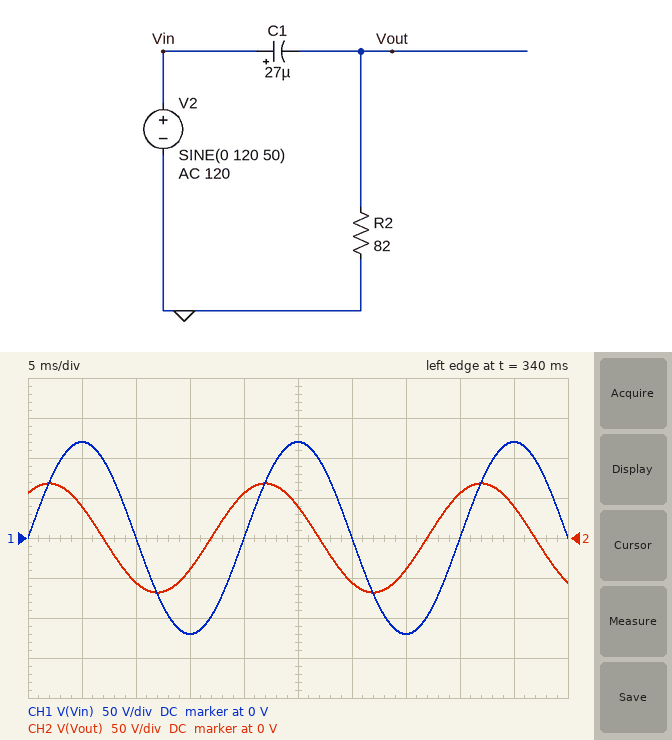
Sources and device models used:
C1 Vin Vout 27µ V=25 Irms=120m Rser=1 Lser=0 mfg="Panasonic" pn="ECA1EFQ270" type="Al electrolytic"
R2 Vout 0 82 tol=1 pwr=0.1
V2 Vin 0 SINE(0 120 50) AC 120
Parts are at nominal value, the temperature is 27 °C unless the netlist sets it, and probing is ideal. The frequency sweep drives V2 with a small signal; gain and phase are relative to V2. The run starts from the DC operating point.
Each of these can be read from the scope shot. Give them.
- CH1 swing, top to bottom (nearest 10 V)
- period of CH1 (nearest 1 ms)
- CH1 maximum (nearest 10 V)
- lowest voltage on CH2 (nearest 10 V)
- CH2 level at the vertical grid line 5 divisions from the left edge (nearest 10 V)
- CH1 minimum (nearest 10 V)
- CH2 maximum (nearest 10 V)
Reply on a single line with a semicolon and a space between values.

240 V; 20 ms; 120 V; -70 V; 40 V; -120 V; 70 V
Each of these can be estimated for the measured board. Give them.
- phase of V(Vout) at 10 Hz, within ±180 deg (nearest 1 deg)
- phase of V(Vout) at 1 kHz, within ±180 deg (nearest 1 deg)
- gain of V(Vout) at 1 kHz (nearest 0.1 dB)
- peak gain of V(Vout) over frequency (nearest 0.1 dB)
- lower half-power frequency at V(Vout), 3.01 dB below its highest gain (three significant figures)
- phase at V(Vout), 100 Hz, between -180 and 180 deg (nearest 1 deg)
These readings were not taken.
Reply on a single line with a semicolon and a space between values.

82 deg; 4 deg; -0.1 dB; -0.1 dB; 71.0 Hz; 35 deg
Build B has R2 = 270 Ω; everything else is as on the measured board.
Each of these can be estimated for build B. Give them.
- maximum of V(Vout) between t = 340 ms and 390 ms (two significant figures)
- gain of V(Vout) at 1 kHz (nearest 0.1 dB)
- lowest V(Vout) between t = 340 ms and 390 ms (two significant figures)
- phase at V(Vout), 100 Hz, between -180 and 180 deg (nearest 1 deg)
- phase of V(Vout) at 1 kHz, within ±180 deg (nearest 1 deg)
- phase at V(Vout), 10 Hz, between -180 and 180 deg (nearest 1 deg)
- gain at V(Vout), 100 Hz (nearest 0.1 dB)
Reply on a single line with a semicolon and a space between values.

110 V; 0 dB; -110 V; 12 deg; 1 deg; 65 deg; -0.2 dB
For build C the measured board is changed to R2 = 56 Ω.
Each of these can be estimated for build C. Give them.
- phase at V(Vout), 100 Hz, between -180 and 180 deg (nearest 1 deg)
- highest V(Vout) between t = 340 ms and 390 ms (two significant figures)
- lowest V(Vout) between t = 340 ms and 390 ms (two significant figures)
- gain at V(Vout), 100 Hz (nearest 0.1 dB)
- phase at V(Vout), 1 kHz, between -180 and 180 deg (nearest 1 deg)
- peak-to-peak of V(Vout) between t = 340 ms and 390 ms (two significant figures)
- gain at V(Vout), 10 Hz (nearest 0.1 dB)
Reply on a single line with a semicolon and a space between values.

46 deg; 51 V; -51 V; -3.3 dB; 6 deg; 100 V; -20.5 dB
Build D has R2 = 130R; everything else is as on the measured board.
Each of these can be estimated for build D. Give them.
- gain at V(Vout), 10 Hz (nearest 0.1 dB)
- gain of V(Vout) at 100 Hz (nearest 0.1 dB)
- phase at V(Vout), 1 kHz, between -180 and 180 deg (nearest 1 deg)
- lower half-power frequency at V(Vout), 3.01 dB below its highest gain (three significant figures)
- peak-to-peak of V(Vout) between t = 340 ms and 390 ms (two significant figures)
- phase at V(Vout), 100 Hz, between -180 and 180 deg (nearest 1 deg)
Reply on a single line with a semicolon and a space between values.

-13.3 dB; -0.9 dB; 3 deg; 45.0 Hz; 180 V; 24 deg
